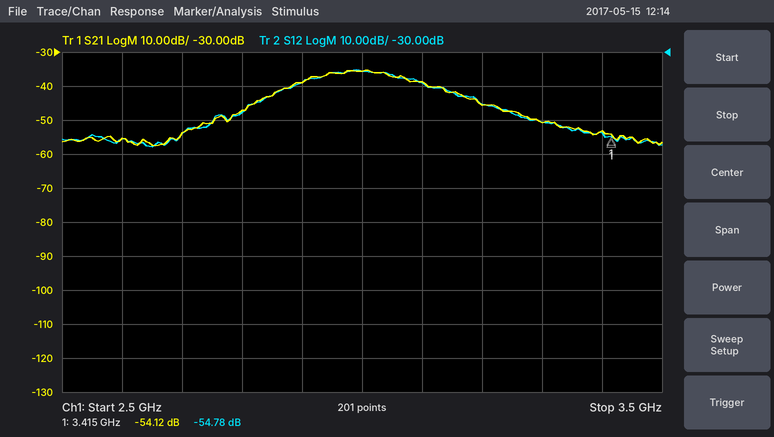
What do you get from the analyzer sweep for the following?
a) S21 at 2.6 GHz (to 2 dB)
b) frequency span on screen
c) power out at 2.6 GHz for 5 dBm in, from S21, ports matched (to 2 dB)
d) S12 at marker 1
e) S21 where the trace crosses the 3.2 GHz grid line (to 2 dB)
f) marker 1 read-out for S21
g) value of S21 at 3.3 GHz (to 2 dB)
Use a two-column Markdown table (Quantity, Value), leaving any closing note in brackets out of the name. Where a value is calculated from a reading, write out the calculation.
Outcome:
| Quantity | Value |
|---|---|
| S21 at 2.6 GHz | -56 dB |
| frequency span on screen | 1 GHz |
| power out at 2.6 GHz for 5 dBm in, from S21, ports matched | 5 dBm + (-56 dB) = -50 dBm |
| S12 at marker 1 | -54.78 dB |
| S21 where the trace crosses the 3.2 GHz grid line | -46 dB |
| marker 1 read-out for S21 | -54.12 dB |
| value of S21 at 3.3 GHz | -50 dB |
